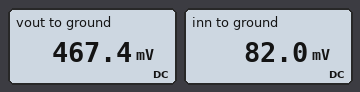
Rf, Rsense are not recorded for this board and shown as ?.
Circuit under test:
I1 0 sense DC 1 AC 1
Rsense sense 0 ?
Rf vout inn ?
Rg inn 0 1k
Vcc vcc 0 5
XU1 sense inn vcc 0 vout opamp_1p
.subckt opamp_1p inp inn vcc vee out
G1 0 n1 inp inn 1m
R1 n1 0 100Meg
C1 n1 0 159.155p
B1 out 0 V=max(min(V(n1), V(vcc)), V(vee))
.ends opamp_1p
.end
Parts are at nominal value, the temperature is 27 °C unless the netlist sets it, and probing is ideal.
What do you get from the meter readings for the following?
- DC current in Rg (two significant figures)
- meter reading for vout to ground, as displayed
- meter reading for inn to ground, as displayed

82 µA
467.4 mV
82.0 mV
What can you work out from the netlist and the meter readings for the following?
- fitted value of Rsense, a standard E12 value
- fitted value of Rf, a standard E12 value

0.082 Ω
4.7 kΩ
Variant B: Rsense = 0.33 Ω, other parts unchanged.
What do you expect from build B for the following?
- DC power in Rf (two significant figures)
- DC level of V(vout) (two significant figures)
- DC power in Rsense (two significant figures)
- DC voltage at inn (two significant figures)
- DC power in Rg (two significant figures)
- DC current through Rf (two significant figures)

510 µW
1.9 V
330 mW
330 mV
110 µW
330 µA
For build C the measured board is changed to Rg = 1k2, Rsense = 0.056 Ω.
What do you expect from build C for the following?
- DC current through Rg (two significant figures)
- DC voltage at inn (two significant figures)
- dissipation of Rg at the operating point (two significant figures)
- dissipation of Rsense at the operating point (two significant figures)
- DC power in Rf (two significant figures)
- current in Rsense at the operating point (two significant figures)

47 µA
56 mV
2.6 µW
56 mW
10 µW
1.0 A
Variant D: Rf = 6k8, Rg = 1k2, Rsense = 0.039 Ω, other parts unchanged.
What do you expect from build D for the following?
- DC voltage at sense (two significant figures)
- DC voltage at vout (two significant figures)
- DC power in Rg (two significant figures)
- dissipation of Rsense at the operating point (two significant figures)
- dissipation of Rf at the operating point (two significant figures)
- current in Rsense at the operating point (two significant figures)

39 mV
260 mV
1.3 µW
39 mW
7.2 µW
1.0 A
